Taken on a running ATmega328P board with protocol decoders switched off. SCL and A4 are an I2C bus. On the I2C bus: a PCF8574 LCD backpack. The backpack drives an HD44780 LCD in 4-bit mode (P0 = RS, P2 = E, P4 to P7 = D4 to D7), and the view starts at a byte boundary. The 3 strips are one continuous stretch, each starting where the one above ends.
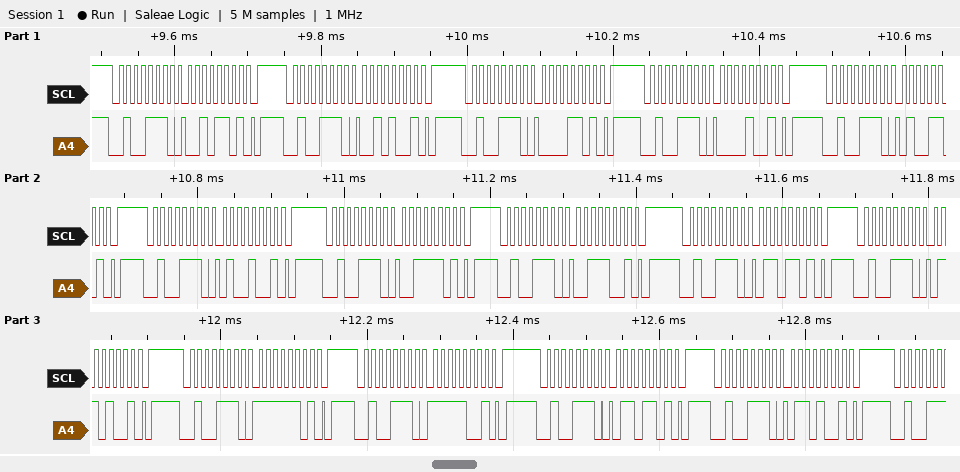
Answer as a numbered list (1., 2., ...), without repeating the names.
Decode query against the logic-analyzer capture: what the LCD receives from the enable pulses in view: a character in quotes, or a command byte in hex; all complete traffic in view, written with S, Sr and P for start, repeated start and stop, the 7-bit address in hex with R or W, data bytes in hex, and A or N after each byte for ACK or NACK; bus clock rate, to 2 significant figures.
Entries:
1. ' ' 'C' 'o'
2. S 27W A 2D A P S 27W A 29 A P S 27W A 0D A P S 27W A 09 A P S 27W A 4D A P S 27W A 49 A P S 27W A 3D A P S 27W A 39 A P S 27W A 6D A P S 27W A 69 A P S 27W A FD A P S 27W A F9 A P S 27W A 6D A P S 27W A 69 A P
3. 100 kHz
